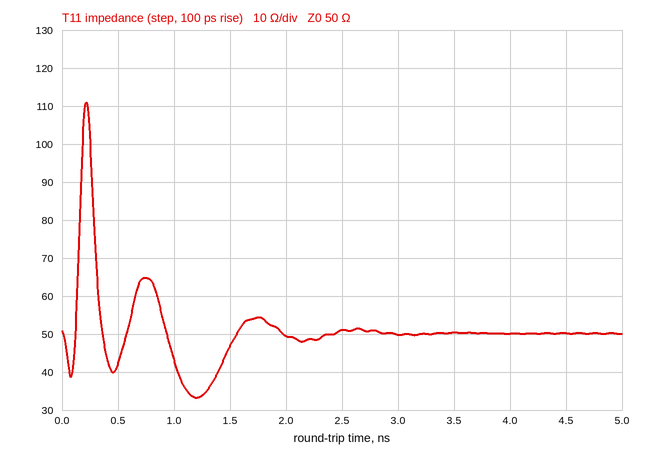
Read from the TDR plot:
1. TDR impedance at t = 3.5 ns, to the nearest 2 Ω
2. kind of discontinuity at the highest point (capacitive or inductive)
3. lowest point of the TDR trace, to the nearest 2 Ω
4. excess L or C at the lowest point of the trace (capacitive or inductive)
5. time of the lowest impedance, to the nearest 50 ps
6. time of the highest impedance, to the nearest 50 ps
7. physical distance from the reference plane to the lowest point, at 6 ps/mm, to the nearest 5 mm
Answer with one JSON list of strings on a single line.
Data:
["50 Ω", "inductive", "34 Ω", "capacitive", "1.20 ns", "200 ps", "100 mm"]
